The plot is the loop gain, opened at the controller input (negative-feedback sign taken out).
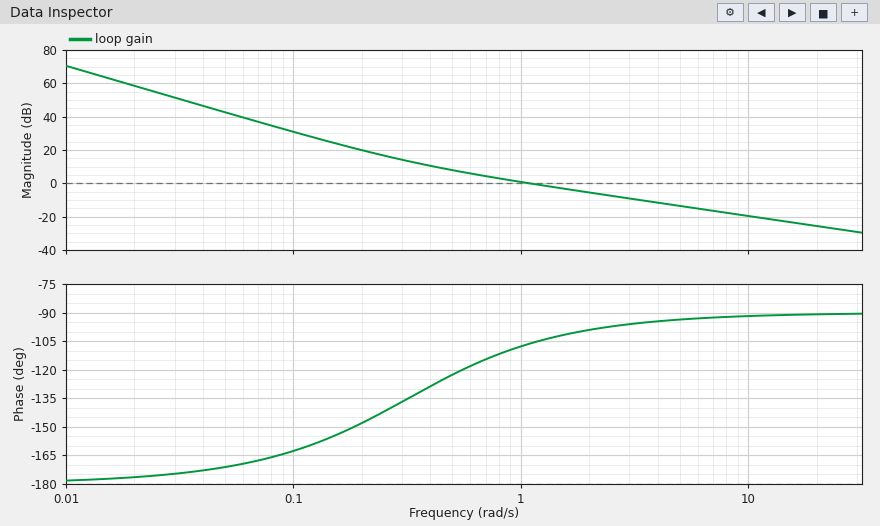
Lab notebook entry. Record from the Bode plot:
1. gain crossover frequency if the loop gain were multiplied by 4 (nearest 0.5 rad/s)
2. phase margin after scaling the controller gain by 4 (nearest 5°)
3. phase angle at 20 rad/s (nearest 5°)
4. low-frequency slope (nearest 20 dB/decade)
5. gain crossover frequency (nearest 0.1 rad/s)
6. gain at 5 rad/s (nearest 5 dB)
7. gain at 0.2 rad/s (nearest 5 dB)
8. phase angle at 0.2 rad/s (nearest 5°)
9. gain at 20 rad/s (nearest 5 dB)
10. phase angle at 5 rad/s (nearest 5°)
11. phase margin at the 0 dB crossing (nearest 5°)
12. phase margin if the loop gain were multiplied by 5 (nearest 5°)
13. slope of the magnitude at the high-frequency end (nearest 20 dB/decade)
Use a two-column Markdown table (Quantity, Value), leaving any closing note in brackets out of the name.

| Quantity | Value |
|---|---|
| gain crossover frequency if the loop gain were multiplied by 4 | 4.0 rad/s |
| phase margin after scaling the controller gain by 4 | 85° |
| phase angle at 20 rad/s | -90° |
| low-frequency slope | -40 dB/decade |
| gain crossover frequency | 1.1 rad/s |
| gain at 5 rad/s | -15 dB |
| gain at 0.2 rad/s | 20 dB |
| phase angle at 0.2 rad/s | -150° |
| gain at 20 rad/s | -25 dB |
| phase angle at 5 rad/s | -95° |
| phase margin at the 0 dB crossing | 75° |
| phase margin if the loop gain were multiplied by 5 | 85° |
| slope of the magnitude at the high-frequency end | -20 dB/decade |
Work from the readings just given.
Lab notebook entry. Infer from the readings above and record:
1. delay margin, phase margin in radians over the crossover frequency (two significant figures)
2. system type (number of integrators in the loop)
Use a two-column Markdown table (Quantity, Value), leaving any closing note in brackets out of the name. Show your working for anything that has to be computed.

| Quantity | Value |
|---|---|
| delay margin, phase margin in radians over the crossover frequency | 75 × π / 180 / 1.1 = 1.2 s |
| system type | 2 |
